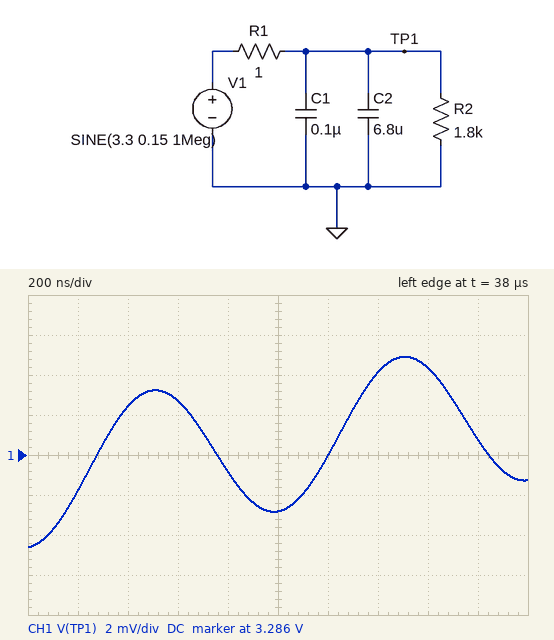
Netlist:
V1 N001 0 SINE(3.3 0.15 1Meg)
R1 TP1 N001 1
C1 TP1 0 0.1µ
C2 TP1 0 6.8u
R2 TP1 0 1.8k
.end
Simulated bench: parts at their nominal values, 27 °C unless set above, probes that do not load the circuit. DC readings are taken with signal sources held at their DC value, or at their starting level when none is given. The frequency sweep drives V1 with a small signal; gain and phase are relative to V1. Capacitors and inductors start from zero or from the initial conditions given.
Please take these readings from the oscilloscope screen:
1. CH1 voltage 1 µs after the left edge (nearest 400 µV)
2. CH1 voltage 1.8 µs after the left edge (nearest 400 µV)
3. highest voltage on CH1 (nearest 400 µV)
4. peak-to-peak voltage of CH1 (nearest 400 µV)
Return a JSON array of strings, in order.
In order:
["3.2832 V", "3.2868 V", "3.2908 V", "9.6 mV"]
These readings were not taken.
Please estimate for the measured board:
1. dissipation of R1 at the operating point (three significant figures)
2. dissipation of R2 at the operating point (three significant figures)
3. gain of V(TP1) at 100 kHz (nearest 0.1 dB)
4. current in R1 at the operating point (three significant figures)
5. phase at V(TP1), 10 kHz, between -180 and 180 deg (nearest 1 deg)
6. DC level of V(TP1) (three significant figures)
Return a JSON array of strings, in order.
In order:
["3.36 µW", "6.04 mW", "-13.0 dB", "1.83 mA", "-23 deg", "3.30 V"]
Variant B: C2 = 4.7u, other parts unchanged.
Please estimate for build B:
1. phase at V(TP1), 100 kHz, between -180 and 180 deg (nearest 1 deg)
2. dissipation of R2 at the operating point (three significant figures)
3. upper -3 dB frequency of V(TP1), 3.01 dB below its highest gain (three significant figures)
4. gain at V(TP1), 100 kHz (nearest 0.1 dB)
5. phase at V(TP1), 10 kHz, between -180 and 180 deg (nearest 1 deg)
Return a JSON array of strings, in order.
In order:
["-72 deg", "6.04 mW", "33.2 kHz", "-10.0 dB", "-17 deg"]
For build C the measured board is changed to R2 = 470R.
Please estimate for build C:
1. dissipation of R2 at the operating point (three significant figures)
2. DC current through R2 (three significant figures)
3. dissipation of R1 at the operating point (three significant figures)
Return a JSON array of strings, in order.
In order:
["23.1 mW", "7.01 mA", "49.1 µW"]
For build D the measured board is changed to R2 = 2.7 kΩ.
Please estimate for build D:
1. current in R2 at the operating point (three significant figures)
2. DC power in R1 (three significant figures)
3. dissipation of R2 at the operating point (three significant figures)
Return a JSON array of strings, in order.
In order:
["1.22 mA", "1.49 µW", "4.03 mW"]
